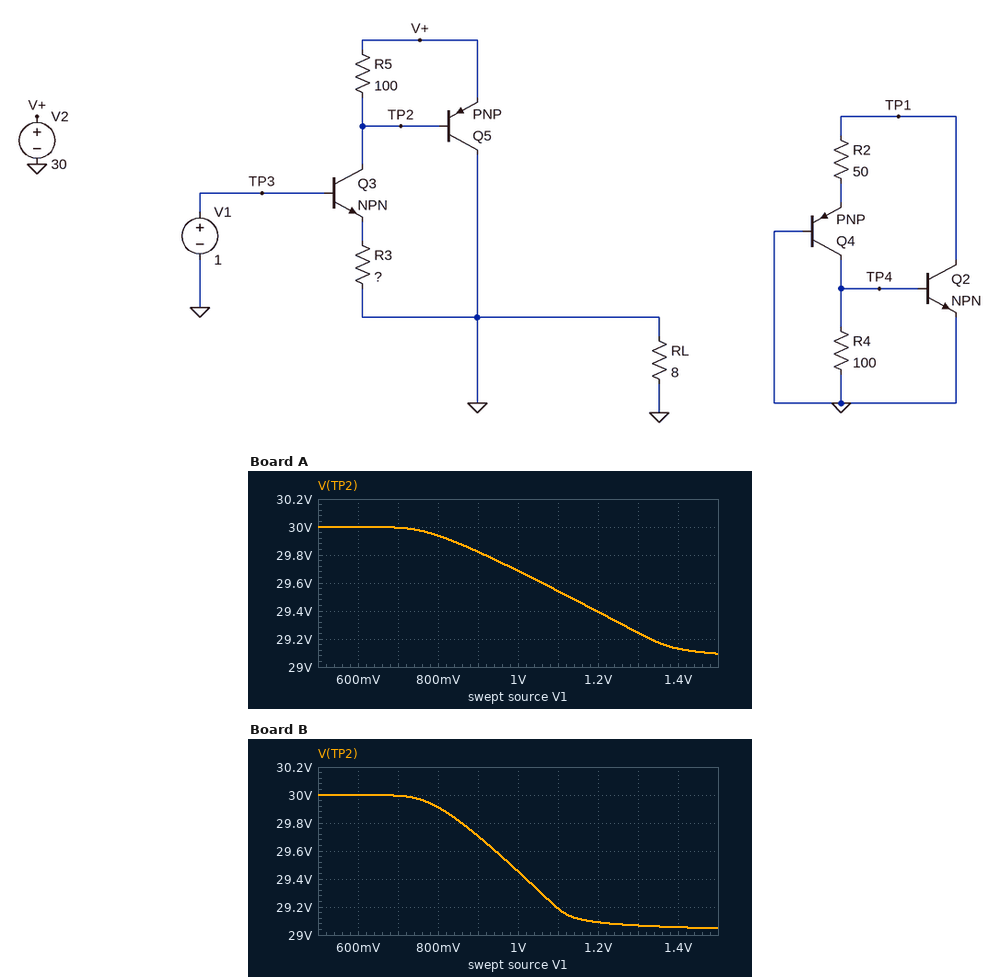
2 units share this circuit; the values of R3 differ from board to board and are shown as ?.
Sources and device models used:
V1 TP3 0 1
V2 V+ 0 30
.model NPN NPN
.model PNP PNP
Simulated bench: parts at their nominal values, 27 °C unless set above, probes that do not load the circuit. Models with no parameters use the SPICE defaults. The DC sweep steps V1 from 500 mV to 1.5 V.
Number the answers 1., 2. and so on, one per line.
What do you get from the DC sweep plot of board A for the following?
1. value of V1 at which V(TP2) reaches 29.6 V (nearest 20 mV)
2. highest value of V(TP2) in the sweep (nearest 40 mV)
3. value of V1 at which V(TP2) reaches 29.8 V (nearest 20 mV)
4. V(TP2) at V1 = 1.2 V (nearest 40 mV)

1. 1.06 V
2. 30.00 V
3. 920 mV
4. 29.40 V
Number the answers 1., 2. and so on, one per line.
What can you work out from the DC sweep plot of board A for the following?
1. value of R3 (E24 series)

1. 62 Ω
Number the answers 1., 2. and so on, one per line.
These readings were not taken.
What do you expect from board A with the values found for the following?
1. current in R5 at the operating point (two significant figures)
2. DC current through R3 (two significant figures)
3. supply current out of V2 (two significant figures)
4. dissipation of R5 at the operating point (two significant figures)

1. 3.1 mA
2. 3.2 mA
3. 3.1 mA
4. 980 µW
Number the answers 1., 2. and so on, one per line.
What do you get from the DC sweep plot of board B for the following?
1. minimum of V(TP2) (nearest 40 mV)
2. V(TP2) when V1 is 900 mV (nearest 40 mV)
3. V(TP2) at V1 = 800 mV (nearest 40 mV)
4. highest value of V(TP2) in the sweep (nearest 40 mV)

1. 29.04 V
2. 29.72 V
3. 29.92 V
4. 30.00 V
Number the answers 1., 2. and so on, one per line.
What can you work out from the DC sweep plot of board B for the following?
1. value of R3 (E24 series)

1. 33 Ω
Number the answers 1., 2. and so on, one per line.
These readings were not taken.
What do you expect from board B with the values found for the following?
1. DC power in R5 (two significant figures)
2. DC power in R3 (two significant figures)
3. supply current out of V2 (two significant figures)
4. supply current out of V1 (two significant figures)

1. 3.0 mW
2. 1.0 mW
3. 5.5 mA
4. 55 µA
